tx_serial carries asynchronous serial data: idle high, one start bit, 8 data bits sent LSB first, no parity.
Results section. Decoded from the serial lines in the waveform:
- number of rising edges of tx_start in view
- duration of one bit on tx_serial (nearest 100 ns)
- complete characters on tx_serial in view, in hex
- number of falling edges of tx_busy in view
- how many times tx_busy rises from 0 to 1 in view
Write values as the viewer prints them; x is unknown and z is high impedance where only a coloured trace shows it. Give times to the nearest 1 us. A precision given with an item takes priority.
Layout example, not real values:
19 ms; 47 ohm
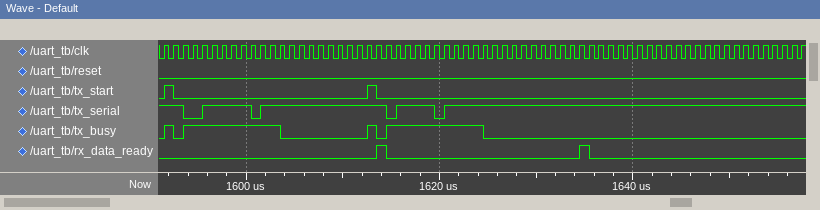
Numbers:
2; 1000 ns; BE, EF; 4; 4
